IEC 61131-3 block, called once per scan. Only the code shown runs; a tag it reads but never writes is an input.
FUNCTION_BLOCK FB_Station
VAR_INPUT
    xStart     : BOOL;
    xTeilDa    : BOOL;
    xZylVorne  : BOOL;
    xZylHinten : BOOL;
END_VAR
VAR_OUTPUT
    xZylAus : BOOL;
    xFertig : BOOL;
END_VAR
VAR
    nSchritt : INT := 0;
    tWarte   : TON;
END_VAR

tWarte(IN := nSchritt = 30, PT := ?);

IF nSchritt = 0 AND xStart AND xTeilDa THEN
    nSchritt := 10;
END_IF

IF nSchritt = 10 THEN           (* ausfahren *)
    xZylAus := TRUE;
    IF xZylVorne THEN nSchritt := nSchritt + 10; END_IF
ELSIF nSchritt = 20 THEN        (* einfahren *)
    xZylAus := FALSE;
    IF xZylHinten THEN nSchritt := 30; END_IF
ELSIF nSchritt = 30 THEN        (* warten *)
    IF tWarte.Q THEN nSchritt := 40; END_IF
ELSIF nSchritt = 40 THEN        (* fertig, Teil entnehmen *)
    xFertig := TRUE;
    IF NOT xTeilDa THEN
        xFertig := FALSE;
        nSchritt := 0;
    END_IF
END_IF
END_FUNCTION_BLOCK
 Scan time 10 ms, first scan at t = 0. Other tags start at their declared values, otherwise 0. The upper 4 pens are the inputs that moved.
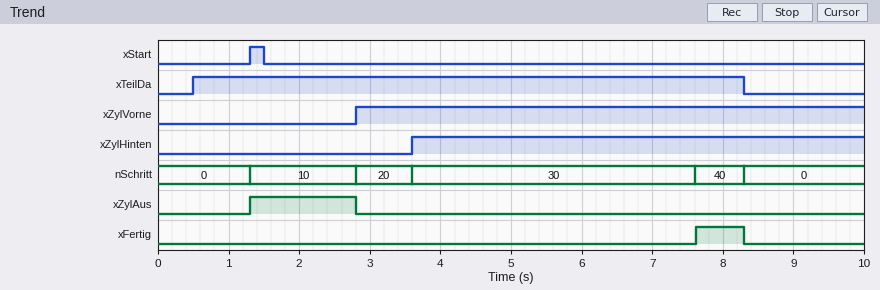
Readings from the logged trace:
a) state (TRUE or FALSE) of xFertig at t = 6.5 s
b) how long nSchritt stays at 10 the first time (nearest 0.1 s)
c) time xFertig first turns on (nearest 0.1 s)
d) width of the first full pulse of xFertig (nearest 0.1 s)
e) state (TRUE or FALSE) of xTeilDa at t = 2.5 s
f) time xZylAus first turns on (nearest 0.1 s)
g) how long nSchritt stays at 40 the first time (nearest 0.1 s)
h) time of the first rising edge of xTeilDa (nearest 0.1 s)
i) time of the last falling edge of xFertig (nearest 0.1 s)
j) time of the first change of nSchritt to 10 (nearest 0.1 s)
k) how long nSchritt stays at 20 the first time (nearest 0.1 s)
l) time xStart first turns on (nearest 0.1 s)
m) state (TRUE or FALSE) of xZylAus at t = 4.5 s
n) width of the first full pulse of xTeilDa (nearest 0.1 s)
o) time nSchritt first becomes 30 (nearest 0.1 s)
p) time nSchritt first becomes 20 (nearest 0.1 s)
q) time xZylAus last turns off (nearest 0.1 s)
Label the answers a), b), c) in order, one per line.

a) FALSE
b) 1.5 s
c) 7.6 s
d) 0.7 s
e) TRUE
f) 1.3 s
g) 0.7 s
h) 0.5 s
i) 8.3 s
j) 1.3 s
k) 0.8 s
l) 1.3 s
m) FALSE
n) 7.8 s
o) 3.6 s
p) 2.8 s
q) 2.8 s
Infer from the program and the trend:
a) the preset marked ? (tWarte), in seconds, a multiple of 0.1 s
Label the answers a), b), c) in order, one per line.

a) 4.0 s
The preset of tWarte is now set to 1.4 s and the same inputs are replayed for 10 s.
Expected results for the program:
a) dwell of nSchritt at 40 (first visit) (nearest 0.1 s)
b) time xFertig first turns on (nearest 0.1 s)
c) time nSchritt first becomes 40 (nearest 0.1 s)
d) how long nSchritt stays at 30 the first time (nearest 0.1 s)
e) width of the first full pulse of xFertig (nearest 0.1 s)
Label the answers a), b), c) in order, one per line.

a) 3.3 s
b) 5.0 s
c) 5.0 s
d) 1.4 s
e) 3.3 s
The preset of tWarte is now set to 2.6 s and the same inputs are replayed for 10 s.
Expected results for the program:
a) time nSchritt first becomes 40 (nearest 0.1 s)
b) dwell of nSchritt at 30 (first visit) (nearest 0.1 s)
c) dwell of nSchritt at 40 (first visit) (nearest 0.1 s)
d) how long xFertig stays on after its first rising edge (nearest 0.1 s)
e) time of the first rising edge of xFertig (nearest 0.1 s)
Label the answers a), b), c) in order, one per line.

a) 6.2 s
b) 2.6 s
c) 2.1 s
d) 2.1 s
e) 6.2 s
